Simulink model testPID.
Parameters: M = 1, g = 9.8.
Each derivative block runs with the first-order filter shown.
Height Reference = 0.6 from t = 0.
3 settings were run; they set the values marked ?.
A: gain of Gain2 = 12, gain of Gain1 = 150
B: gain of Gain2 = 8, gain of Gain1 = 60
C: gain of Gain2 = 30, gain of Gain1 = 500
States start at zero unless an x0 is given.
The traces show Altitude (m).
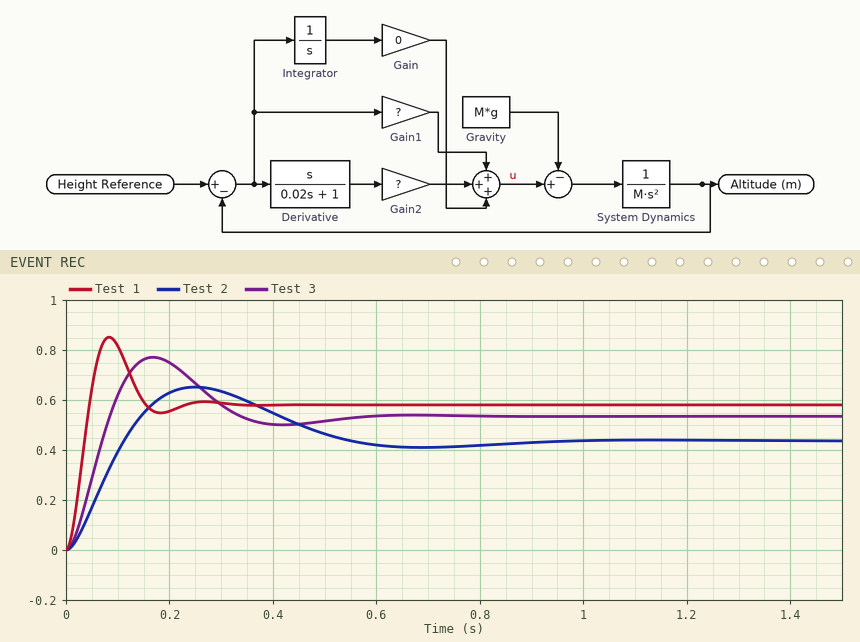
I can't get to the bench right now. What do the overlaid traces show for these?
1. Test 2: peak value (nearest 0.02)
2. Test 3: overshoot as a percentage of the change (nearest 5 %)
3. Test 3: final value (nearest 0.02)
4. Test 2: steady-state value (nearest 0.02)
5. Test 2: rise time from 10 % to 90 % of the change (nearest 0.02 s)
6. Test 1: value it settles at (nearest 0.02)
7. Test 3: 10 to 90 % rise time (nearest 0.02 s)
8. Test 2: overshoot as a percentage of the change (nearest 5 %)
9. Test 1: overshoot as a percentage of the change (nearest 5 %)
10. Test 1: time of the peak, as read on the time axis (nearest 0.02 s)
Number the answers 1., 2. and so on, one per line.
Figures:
1. 0.66
2. 45 %
3. 0.54
4. 0.44
5. 0.08 s
6. 0.58
7. 0.06 s
8. 50 %
9. 45 %
10. 0.08 s
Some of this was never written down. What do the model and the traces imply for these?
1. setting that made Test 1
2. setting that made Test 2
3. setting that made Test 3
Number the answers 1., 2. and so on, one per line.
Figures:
1. C
2. B
3. A
